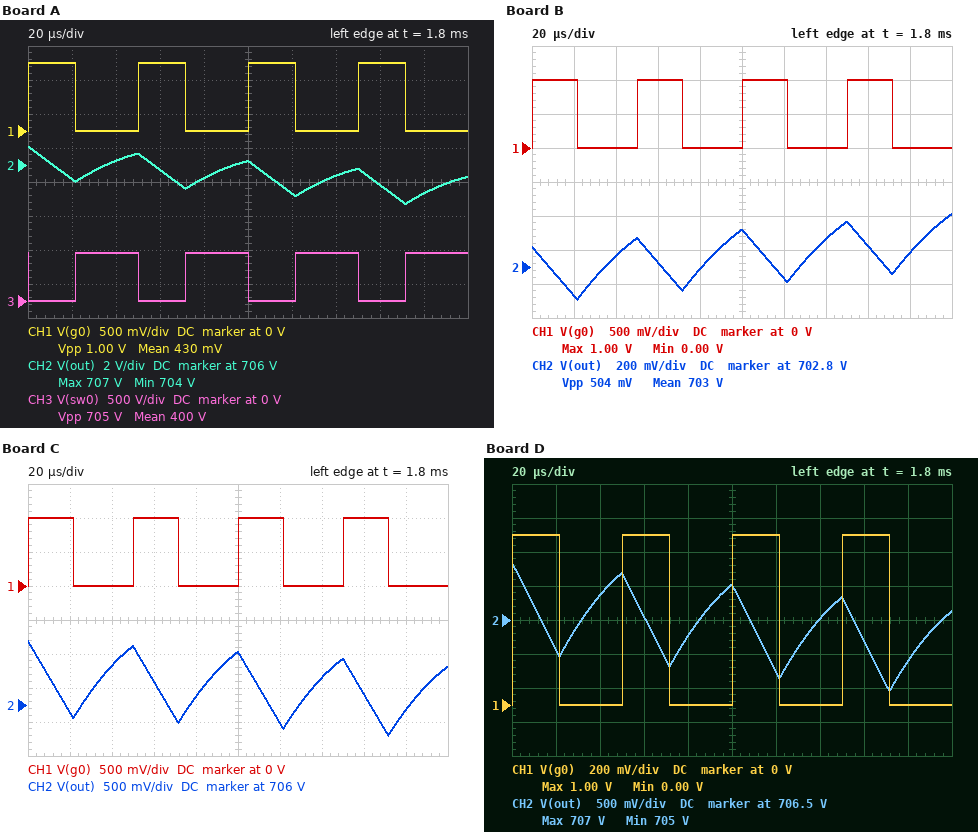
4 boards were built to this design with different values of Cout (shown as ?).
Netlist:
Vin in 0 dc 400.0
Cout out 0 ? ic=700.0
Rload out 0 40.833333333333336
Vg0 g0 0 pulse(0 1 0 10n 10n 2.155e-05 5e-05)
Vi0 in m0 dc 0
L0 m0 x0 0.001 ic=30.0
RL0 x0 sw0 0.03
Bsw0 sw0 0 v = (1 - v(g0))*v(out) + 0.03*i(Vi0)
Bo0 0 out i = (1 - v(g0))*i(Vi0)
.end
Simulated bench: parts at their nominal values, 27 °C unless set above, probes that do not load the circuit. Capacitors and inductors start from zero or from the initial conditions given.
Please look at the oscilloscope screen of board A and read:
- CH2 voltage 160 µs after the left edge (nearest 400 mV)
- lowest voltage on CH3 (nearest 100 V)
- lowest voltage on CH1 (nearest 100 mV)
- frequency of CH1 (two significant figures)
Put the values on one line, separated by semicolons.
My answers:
704.8 V; 0 V; 0 V; 20 kHz
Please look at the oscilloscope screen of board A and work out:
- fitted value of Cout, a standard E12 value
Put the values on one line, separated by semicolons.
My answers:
180 µF
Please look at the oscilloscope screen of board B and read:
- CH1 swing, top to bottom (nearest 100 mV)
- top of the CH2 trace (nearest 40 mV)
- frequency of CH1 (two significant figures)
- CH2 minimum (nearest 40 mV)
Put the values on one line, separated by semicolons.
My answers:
1.0 V; 703.12 V; 20 kHz; 702.60 V
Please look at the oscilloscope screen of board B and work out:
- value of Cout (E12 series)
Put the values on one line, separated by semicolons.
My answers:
1.2 mF
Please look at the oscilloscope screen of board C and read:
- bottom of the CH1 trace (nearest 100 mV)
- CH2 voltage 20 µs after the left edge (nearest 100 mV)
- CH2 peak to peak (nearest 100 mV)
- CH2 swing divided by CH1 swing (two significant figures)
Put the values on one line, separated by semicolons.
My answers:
0 V; 705.9 V; 1.4 V; 1.4
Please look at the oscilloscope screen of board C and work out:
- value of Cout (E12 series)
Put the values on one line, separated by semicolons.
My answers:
330 µF
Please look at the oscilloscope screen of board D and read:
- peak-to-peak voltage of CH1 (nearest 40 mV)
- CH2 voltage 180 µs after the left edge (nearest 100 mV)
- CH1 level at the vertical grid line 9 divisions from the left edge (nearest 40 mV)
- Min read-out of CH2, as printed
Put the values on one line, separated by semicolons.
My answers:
1.00 V; 705.9 V; 0 V; 705 V
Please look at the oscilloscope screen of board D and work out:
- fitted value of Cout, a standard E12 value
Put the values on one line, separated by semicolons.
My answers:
270 µF
